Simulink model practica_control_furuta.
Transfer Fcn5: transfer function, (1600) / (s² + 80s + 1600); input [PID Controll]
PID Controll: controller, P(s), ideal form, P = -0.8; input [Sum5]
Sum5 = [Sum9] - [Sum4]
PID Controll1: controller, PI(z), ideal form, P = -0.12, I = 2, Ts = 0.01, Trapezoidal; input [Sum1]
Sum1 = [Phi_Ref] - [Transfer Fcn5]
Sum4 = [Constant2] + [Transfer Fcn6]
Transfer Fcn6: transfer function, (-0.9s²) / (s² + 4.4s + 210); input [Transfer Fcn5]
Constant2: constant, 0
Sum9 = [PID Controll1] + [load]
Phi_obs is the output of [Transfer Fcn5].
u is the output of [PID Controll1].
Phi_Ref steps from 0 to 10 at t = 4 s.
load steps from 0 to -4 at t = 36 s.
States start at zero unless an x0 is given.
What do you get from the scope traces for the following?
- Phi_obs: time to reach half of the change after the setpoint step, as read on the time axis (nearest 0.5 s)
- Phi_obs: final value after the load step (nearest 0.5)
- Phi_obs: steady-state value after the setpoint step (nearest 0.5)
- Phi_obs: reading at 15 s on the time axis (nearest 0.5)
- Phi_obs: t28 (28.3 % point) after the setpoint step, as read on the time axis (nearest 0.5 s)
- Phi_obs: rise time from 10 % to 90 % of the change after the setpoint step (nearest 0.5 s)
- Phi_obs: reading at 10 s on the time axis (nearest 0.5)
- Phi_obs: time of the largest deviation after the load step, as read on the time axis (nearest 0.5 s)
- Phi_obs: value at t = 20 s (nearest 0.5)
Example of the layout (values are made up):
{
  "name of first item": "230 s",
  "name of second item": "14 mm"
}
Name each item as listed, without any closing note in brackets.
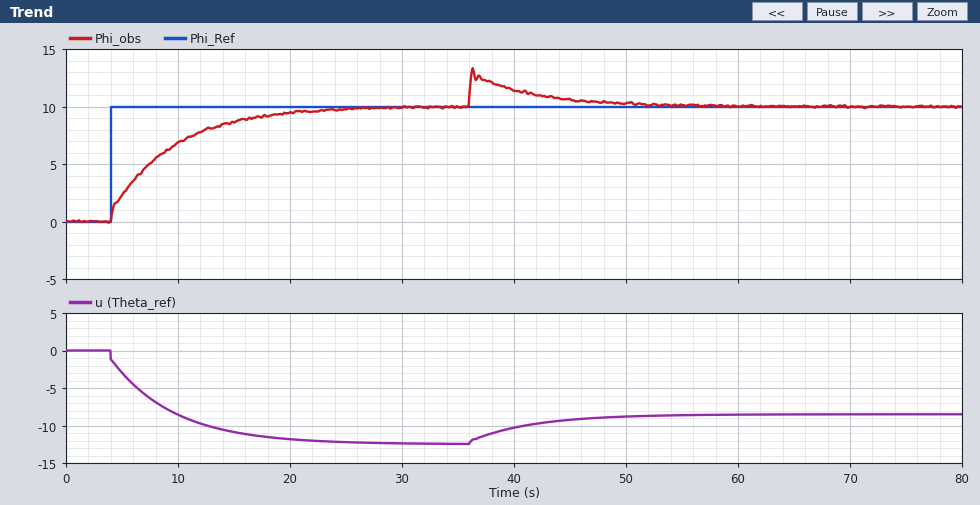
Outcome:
{
  "Phi_obs: time to reach half of the change after the setpoint step, as read on the time axis": "7.5 s",
  "Phi_obs: final value after the load step": "10.0",
  "Phi_obs: steady-state value after the setpoint step": "10.0",
  "Phi_obs: reading at 15 s on the time axis": "8.5",
  "Phi_obs: t28 (28.3 % point) after the setpoint step, as read on the time axis": "5.5 s",
  "Phi_obs: rise time from 10 % to 90 % of the change after the setpoint step": "12.5 s",
  "Phi_obs: reading at 10 s on the time axis": "7.0",
  "Phi_obs: time of the largest deviation after the load step, as read on the time axis": "36.5 s",
  "Phi_obs: value at t = 20 s": "9.5"
}
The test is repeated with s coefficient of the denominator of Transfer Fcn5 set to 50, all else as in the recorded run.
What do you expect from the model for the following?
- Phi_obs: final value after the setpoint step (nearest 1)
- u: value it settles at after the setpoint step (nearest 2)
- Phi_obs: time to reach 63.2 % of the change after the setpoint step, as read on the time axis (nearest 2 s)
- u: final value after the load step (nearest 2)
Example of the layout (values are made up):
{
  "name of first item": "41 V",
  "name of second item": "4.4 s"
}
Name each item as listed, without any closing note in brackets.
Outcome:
{
  "Phi_obs: final value after the setpoint step": "10",
  "u: value it settles at after the setpoint step": "-12",
  "Phi_obs: time to reach 63.2 % of the change after the setpoint step, as read on the time axis": "10 s",
  "u: final value after the load step": "-8"
}
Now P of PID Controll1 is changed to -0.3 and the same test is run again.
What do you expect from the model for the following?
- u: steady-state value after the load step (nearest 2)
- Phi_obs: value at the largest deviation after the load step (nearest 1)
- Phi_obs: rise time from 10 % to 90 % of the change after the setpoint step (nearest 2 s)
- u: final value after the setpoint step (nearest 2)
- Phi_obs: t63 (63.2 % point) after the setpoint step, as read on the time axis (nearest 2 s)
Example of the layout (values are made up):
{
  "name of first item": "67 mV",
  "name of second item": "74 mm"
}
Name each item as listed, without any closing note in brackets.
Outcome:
{
  "u: steady-state value after the load step": "-8",
  "Phi_obs: value at the largest deviation after the load step": "13",
  "Phi_obs: rise time from 10 % to 90 % of the change after the setpoint step": "6 s",
  "u: final value after the setpoint step": "-12",
  "Phi_obs: t63 (63.2 % point) after the setpoint step, as read on the time axis": "6 s"
}
